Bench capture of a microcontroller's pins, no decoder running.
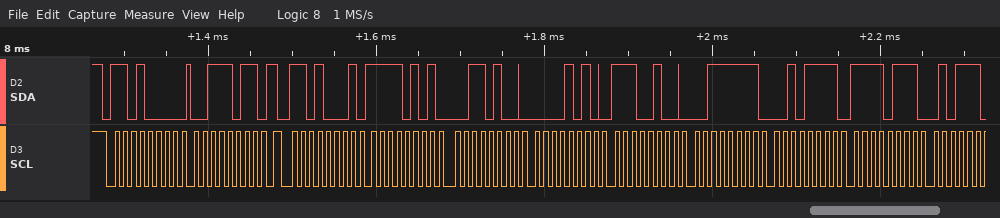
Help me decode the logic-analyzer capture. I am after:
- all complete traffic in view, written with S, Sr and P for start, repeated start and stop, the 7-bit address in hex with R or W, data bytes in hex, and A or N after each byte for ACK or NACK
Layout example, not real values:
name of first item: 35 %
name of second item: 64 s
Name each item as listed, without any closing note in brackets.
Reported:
all complete traffic in view, written with S, Sr and P for start, repeated start and stop, the 7-bit address in hex with R or W, data bytes in hex, and A or N after each byte for ACK or NACK: S 68W A 3B A Sr 68R A F5 A 34 A 0A A E4 A 3F A 2F A F7 A
